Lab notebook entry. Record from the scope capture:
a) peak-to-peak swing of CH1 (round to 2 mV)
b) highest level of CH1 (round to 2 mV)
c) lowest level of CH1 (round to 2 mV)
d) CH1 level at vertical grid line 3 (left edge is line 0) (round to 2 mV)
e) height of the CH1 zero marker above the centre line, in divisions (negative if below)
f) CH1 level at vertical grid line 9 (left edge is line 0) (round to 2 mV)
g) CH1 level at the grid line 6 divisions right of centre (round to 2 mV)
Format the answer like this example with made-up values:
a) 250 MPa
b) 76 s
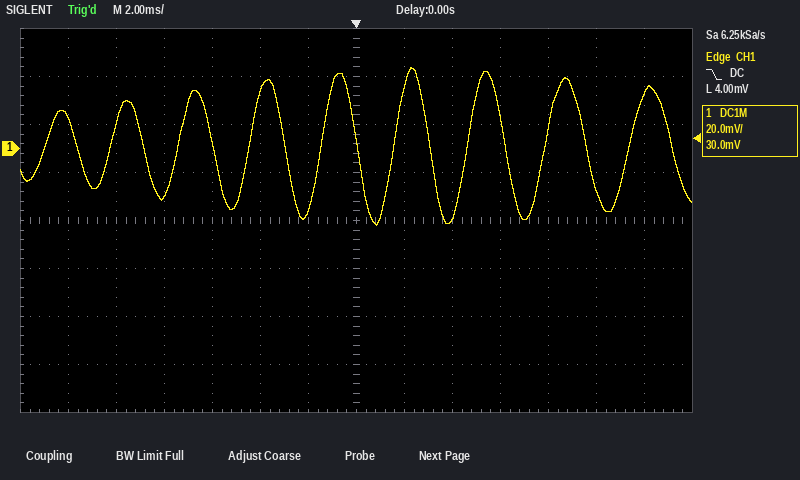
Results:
a) 66 mV
b) 34 mV
c) -32 mV
d) -20 mV
e) +1.5 div
f) -30 mV
g) 22 mV
